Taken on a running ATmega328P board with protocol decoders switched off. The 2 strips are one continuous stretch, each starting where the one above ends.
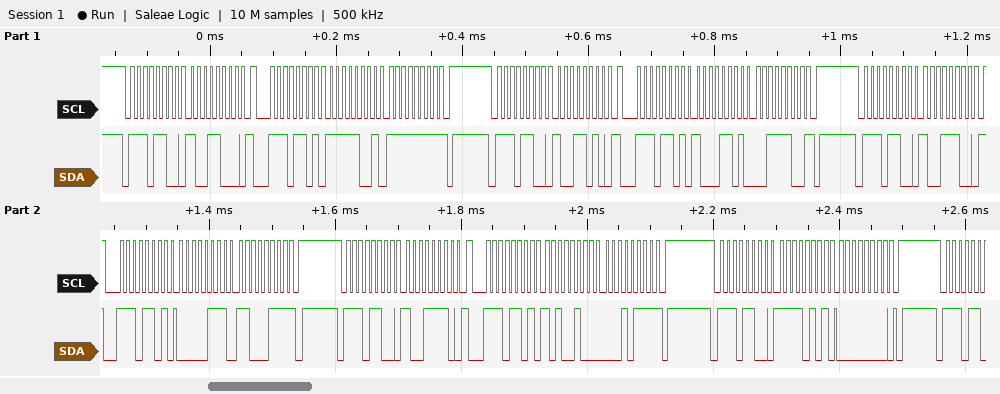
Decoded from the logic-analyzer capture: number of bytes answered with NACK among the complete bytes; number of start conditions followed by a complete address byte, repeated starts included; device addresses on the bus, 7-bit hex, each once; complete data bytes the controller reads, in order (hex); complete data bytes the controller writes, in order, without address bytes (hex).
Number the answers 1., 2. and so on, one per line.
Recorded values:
1. 4
2. 9
3. 0x76
4. F9 FF 8D 3C 07 C7 A4 17
5. 98 9A 9C 9E F5 00
